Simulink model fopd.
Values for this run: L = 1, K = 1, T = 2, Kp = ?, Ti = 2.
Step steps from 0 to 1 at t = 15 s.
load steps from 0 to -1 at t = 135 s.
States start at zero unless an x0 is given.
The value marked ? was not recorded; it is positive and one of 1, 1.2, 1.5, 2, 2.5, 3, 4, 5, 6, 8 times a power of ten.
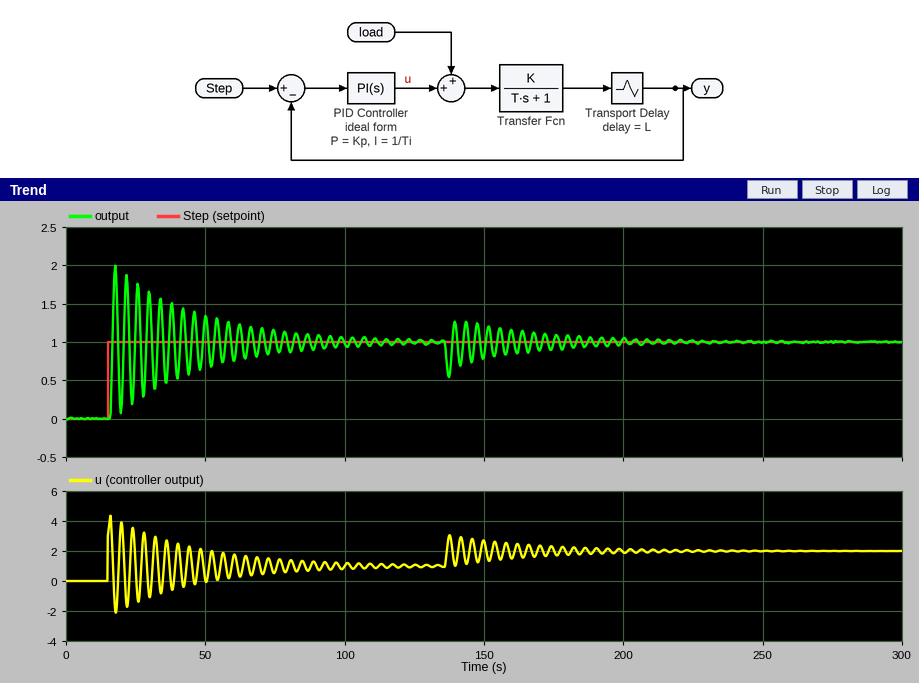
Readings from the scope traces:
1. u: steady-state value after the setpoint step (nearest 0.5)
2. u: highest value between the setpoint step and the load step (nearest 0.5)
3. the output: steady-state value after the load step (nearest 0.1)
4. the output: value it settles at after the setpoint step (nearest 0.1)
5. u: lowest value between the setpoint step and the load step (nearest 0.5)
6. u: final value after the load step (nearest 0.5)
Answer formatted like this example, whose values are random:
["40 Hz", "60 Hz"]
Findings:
["1.0", "4.5", "1.0", "1.0", "-2.0", "2.0"]
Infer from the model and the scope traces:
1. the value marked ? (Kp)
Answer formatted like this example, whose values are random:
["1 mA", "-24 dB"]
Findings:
["3"]
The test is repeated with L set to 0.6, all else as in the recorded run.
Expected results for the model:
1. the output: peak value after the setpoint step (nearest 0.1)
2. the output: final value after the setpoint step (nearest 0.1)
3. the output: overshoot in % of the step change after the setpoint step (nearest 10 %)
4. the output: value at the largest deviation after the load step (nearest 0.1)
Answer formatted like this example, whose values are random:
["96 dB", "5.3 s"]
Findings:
["1.4", "1.0", "40 %", "0.7"]
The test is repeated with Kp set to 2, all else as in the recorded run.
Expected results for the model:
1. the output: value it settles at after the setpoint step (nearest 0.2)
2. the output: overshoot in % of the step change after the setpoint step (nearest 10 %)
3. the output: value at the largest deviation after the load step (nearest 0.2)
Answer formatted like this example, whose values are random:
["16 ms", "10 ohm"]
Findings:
["1.0", "50 %", "0.6"]
